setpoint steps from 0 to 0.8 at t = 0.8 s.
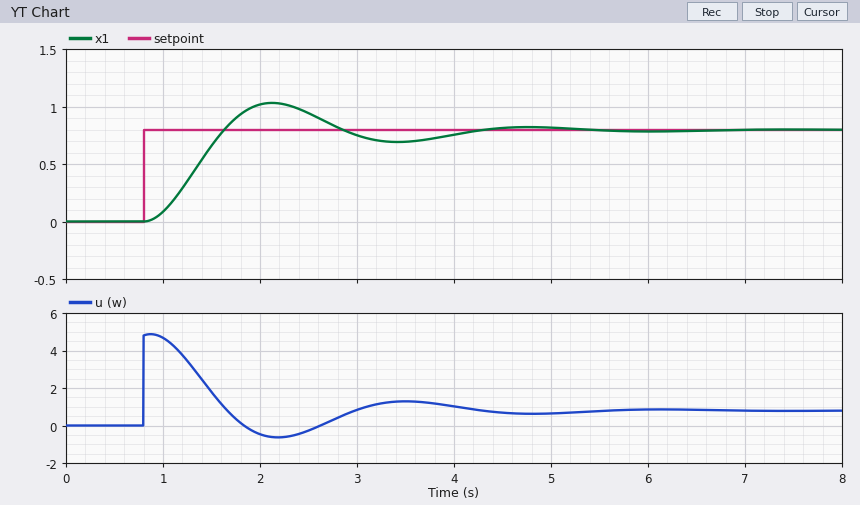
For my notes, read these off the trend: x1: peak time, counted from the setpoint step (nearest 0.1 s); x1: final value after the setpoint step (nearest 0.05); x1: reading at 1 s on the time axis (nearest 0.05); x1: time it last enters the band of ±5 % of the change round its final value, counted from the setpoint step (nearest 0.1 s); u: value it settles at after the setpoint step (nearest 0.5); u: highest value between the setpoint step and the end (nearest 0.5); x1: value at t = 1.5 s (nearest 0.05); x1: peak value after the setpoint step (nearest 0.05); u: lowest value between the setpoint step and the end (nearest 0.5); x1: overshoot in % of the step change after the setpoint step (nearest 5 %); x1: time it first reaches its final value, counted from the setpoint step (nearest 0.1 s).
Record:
1.3 s
0.80
0.10
3.2 s
1.0
5.0
0.65
1.05
-0.5
30 %
0.8 s
